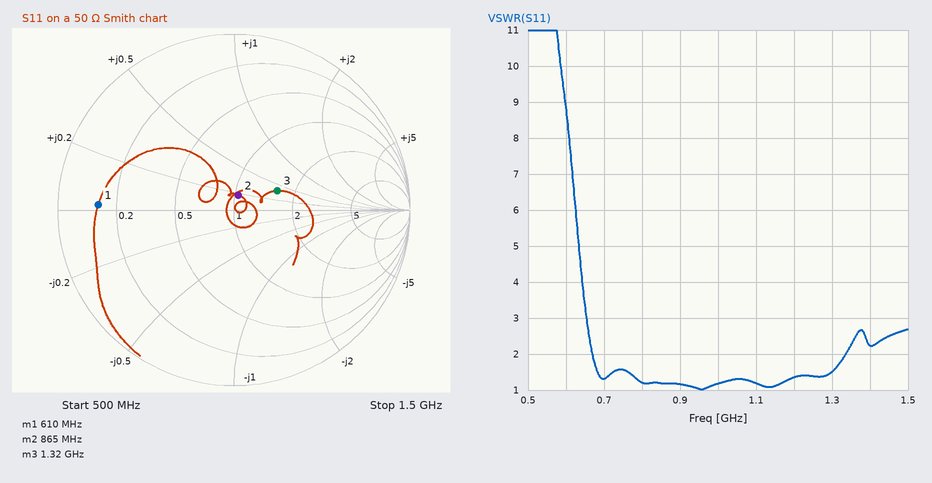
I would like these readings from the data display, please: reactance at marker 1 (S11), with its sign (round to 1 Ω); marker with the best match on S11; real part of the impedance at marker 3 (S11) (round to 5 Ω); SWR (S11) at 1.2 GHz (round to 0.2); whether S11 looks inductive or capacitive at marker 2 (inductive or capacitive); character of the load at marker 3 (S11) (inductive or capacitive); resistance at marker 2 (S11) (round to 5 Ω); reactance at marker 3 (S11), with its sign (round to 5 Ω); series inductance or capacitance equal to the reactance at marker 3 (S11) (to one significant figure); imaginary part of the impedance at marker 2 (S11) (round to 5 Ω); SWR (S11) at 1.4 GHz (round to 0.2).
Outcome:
+1 Ω
marker 2
80 Ω
1.4
inductive
inductive
50 Ω
+20 Ω
2 nH
+10 Ω
2.2
